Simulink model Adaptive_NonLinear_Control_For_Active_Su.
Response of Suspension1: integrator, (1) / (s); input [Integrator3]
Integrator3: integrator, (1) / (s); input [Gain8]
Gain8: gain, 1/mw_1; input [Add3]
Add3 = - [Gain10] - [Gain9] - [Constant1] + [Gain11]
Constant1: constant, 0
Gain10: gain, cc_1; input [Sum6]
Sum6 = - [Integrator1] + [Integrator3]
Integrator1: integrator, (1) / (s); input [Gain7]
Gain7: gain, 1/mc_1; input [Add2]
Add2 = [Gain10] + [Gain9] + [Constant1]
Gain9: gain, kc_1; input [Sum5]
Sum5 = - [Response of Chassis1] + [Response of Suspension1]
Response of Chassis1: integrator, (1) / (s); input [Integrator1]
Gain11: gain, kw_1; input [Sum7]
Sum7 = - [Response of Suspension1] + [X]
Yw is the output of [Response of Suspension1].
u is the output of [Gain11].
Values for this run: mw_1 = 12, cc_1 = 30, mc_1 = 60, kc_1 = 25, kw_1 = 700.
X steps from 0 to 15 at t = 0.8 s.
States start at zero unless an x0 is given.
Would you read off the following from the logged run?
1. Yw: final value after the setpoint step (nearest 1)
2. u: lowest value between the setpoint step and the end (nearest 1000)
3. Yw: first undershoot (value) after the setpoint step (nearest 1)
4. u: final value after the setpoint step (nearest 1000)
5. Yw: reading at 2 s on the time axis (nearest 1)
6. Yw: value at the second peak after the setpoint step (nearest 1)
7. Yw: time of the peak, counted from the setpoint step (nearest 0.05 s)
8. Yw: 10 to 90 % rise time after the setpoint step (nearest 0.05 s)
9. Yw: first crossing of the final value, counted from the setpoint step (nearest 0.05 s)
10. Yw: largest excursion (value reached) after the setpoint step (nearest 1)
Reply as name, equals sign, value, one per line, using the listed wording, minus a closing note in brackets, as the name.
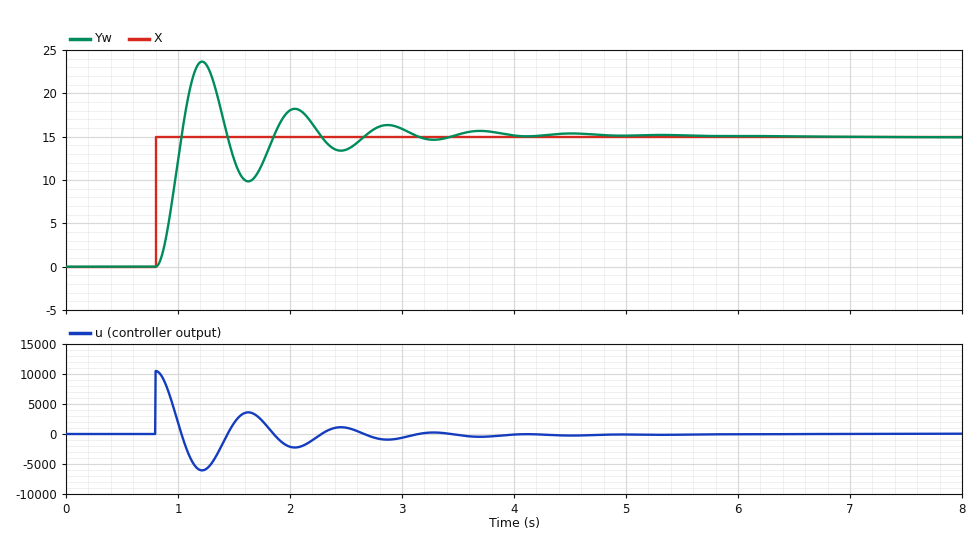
Yw: final value after the setpoint step = 15
u: lowest value between the setpoint step and the end = -6000
Yw: first undershoot (value) after the setpoint step = 10
u: final value after the setpoint step = 0
Yw: reading at 2 s on the time axis = 18
Yw: value at the second peak after the setpoint step = 18
Yw: time of the peak, counted from the setpoint step = 0.40 s
Yw: 10 to 90 % rise time after the setpoint step = 0.15 s
Yw: first crossing of the final value, counted from the setpoint step = 0.25 s
Yw: largest excursion (value reached) after the setpoint step = 24
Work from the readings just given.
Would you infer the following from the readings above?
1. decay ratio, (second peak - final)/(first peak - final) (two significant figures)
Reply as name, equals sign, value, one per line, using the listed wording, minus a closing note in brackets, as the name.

decay ratio, (second peak - final)/(first peak - final) = 0.33
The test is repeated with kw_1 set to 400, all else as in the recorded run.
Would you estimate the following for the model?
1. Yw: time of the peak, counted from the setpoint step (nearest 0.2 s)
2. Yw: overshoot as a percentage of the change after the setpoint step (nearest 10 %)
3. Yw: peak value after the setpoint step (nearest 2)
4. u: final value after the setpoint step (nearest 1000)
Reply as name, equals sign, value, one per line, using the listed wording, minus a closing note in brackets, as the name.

Yw: time of the peak, counted from the setpoint step = 0.6 s
Yw: overshoot as a percentage of the change after the setpoint step = 50 %
Yw: peak value after the setpoint step = 22
u: final value after the setpoint step = 0
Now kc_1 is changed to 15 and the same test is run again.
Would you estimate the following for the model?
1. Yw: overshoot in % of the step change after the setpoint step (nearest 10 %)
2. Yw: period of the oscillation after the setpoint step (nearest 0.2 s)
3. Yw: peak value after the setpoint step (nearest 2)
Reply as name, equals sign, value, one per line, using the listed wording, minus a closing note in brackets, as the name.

Yw: overshoot in % of the step change after the setpoint step = 60 %
Yw: period of the oscillation after the setpoint step = 0.8 s
Yw: peak value after the setpoint step = 24
